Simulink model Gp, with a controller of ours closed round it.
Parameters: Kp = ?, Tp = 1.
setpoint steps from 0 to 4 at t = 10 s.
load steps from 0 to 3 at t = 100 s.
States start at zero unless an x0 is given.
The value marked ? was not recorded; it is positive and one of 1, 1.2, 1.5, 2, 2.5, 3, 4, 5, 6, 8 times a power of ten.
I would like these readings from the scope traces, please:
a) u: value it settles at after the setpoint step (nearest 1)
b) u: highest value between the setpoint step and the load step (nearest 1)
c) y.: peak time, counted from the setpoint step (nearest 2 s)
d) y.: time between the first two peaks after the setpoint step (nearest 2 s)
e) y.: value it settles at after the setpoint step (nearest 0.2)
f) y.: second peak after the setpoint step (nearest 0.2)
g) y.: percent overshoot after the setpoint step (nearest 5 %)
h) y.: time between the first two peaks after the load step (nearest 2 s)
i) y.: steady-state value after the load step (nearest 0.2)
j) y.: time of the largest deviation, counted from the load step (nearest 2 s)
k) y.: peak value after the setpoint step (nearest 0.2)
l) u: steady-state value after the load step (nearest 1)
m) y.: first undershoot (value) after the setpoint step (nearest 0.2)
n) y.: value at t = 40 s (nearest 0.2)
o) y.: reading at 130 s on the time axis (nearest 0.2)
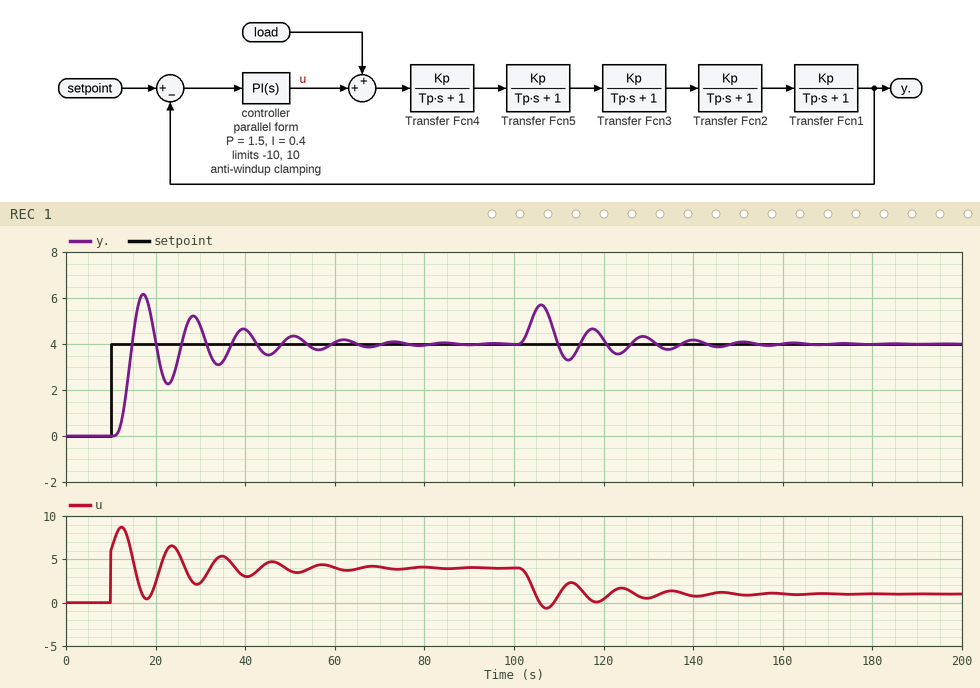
4
9
8 s
12 s
4.0
5.2
55 %
12 s
4.0
6 s
6.2
1
2.2
4.6
4.2
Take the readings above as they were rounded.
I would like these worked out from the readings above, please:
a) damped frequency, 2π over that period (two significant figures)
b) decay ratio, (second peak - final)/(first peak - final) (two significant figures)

0.52 rad/s
0.55
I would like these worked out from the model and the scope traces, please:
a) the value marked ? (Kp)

1
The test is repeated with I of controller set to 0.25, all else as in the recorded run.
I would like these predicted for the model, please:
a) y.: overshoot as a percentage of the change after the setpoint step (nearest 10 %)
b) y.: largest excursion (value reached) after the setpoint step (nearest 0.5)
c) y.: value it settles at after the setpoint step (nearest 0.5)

30 %
5.0
4.0
